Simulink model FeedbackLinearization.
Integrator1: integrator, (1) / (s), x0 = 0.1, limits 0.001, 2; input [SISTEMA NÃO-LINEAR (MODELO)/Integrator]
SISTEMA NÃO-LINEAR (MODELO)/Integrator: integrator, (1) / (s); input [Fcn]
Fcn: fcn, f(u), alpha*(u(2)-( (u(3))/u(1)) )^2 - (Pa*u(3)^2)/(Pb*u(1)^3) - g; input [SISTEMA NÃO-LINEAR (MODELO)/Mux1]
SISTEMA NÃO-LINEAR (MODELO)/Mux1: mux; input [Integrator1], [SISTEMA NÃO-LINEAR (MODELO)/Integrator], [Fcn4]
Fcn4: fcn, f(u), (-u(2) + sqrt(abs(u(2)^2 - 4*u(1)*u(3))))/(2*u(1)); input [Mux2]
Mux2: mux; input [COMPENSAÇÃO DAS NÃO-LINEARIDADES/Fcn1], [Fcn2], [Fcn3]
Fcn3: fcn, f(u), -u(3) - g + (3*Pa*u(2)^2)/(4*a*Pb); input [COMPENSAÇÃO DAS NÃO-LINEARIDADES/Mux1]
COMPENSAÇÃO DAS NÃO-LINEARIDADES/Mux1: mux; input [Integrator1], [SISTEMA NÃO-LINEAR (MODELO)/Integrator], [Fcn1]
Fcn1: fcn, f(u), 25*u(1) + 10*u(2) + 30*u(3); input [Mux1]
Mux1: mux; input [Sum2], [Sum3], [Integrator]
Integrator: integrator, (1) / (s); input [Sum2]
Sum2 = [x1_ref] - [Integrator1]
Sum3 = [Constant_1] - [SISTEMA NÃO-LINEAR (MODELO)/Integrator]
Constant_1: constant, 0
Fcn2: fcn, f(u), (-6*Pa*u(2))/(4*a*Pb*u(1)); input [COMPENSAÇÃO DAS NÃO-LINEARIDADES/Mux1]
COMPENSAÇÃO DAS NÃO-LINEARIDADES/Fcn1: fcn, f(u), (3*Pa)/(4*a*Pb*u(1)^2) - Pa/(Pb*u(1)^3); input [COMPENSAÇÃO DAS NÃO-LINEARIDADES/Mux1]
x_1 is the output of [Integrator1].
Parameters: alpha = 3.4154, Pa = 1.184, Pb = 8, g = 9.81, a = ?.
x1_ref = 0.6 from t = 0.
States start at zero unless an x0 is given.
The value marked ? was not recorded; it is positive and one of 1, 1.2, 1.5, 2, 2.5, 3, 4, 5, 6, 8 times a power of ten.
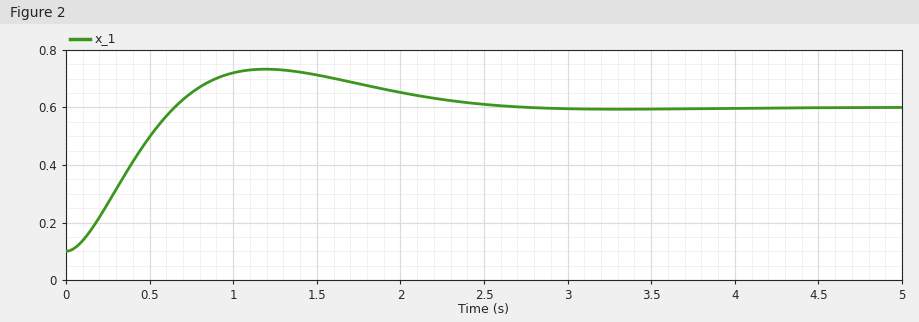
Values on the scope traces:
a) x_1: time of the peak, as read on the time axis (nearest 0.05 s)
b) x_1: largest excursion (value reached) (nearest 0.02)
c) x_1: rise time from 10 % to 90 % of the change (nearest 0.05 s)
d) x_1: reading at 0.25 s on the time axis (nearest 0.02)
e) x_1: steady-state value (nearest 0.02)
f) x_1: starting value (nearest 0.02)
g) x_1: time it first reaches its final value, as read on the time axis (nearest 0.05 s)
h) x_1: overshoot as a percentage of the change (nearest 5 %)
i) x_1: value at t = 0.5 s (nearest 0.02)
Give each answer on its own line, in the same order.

1.20 s
0.74
0.45 s
0.26
0.60
0.10
0.65 s
25 %
0.50
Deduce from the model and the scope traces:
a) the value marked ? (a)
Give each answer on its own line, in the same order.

0.03
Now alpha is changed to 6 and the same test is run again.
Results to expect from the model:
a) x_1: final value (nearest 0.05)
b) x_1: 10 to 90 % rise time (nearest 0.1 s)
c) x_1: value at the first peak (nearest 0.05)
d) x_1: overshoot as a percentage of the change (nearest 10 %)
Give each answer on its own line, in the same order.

0.60
0.3 s
0.80
40 %
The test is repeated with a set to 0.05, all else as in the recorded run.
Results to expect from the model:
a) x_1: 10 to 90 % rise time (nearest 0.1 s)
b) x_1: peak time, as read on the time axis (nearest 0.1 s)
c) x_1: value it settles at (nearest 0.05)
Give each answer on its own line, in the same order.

0.3 s
0.9 s
0.60
